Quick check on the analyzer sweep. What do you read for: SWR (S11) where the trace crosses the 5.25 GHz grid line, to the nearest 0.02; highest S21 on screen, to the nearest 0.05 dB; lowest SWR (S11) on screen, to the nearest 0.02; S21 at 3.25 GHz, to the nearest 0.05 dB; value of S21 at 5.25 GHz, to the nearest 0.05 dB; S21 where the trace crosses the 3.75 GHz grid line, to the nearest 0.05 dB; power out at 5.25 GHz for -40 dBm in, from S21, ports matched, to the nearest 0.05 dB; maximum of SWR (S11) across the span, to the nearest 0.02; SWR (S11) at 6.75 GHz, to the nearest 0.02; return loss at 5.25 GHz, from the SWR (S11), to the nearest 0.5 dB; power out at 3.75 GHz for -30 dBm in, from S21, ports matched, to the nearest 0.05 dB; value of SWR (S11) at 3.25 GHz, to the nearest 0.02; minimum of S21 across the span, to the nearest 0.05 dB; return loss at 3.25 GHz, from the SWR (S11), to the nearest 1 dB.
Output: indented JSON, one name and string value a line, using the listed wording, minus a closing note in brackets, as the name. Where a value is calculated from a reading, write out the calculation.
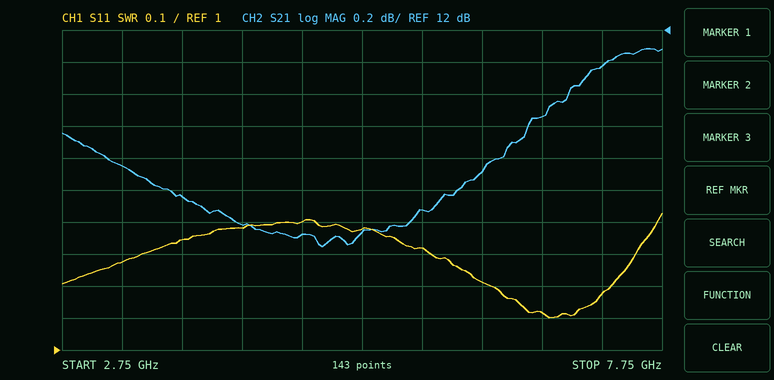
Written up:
{
  "SWR (S11) where the trace crosses the 5.25 GHz grid line, to the nearest 0.02": "1.38",
  "highest S21 on screen, to the nearest 0.05 dB": "11.90 dB",
  "lowest SWR (S11) on screen, to the nearest 0.02": "1.10",
  "S21 at 3.25 GHz, to the nearest 0.05 dB": "11.15 dB",
  "value of S21 at 5.25 GHz, to the nearest 0.05 dB": "10.75 dB",
  "S21 where the trace crosses the 3.75 GHz grid line, to the nearest 0.05 dB": "10.95 dB",
  "power out at 5.25 GHz for -40 dBm in, from S21, ports matched, to the nearest 0.05 dB": "-40 dBm + (10.75 dB) = -29.25 dBm",
  "maximum of SWR (S11) across the span, to the nearest 0.02": "1.42",
  "SWR (S11) at 6.75 GHz, to the nearest 0.02": "1.12",
  "return loss at 5.25 GHz, from the SWR (S11), to the nearest 0.5 dB": "−20 log10((1.38 − 1)/(1.38 + 1)) ≈ 15.9 dB, so 16.0 dB to the nearest 0.5 dB",
  "power out at 3.75 GHz for -30 dBm in, from S21, ports matched, to the nearest 0.05 dB": "-30 dBm + (10.95 dB) = -19.05 dBm",
  "value of SWR (S11) at 3.25 GHz, to the nearest 0.02": "1.28",
  "minimum of S21 across the span, to the nearest 0.05 dB": "10.65 dB",
  "return loss at 3.25 GHz, from the SWR (S11), to the nearest 1 dB": "−20 log10((1.28 − 1)/(1.28 + 1)) ≈ 18 dB"
}
